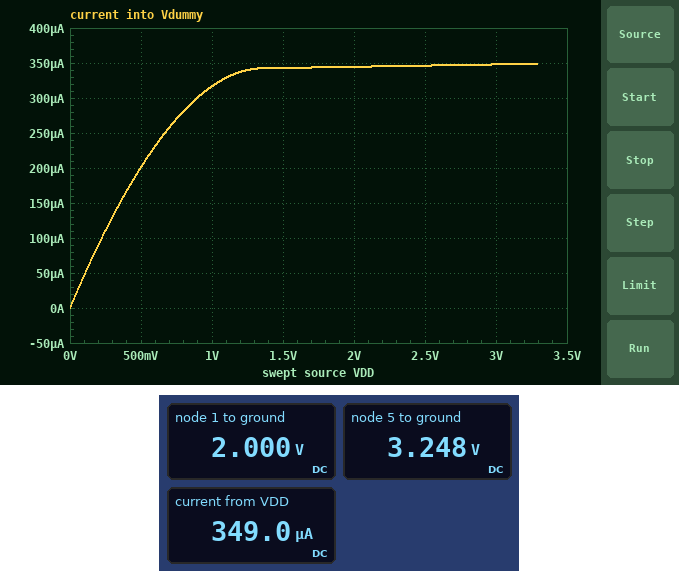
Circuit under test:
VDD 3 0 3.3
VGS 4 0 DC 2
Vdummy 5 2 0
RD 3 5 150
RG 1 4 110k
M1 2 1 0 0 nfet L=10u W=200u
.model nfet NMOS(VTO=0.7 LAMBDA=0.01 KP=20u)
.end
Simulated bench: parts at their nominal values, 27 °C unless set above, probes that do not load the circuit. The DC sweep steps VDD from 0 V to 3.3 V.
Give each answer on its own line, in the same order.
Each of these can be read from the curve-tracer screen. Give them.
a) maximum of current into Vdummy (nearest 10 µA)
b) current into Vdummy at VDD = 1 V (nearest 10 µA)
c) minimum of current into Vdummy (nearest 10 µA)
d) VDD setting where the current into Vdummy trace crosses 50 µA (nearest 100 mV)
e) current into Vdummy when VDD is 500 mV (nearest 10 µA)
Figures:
350 µA
320 µA
0 A
100 mV
200 µA
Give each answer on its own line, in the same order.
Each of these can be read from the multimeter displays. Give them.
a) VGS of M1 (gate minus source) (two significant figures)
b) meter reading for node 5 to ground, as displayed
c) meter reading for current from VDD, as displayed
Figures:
2.0 V
3.248 V
349.0 µA
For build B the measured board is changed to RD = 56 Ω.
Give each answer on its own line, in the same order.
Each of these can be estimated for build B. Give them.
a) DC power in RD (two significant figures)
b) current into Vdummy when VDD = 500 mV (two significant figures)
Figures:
6.8 µW
210 µA
